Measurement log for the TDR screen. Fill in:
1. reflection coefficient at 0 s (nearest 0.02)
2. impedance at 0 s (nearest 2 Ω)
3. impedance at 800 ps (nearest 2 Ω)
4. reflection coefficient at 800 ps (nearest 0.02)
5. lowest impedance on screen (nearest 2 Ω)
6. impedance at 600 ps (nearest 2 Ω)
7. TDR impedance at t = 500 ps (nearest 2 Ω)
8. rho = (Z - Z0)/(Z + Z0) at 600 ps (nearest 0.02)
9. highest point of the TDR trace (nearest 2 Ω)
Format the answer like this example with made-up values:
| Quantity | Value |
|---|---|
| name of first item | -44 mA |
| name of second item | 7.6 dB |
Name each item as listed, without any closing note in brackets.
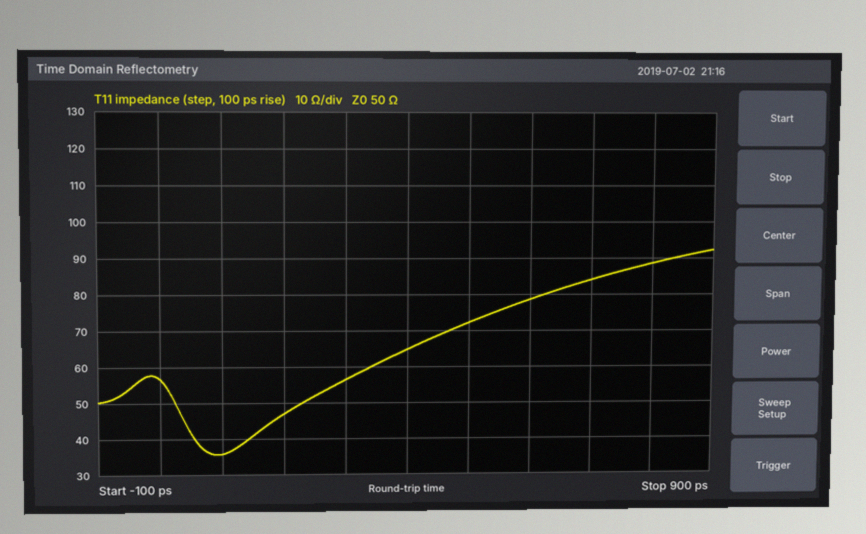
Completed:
| Quantity | Value |
|---|---|
| reflection coefficient at 0 s | +0.06 |
| impedance at 0 s | 56 Ω |
| impedance at 800 ps | 88 Ω |
| reflection coefficient at 800 ps | +0.28 |
| lowest impedance on screen | 36 Ω |
| impedance at 600 ps | 78 Ω |
| TDR impedance at t = 500 ps | 72 Ω |
| rho = (Z - Z0)/(Z + Z0) at 600 ps | +0.22 |
| highest point of the TDR trace | 92 Ω |
